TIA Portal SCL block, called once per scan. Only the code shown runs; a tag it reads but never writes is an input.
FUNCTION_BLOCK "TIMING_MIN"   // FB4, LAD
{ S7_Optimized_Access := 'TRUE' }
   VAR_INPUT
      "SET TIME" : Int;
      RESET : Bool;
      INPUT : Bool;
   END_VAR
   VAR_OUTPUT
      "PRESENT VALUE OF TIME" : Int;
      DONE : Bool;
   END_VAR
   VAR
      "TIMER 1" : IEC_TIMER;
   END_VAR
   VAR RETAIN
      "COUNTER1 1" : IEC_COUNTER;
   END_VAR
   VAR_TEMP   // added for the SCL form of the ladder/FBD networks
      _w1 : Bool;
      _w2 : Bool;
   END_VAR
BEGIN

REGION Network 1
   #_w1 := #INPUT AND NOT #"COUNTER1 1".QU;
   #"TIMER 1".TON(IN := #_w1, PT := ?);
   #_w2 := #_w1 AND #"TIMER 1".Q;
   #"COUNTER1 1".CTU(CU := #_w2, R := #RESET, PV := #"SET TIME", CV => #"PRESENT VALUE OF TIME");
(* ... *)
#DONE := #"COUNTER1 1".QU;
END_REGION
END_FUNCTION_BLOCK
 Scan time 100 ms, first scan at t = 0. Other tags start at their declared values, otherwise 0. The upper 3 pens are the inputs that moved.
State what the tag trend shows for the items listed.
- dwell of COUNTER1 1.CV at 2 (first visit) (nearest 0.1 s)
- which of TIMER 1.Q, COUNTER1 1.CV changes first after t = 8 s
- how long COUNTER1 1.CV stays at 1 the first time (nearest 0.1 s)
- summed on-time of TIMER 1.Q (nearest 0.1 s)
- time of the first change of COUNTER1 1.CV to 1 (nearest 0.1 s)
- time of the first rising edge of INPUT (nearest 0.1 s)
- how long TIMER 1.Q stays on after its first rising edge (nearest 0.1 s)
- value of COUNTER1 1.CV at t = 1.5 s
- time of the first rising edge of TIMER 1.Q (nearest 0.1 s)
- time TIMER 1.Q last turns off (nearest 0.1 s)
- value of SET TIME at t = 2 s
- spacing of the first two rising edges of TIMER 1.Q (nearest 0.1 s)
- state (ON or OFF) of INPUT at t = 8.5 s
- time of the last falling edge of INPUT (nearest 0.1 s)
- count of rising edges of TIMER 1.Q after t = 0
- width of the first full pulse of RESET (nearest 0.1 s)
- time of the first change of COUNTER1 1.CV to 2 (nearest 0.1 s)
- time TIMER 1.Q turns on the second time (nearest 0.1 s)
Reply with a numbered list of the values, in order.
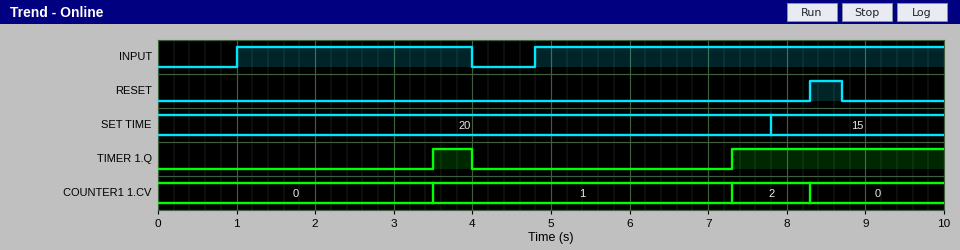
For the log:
1. 1.0 s
2. COUNTER1 1.CV
3. 3.8 s
4. 3.2 s
5. 3.5 s
6. 1.0 s
7. 0.5 s
8. 0
9. 3.5 s
10. 4.0 s
11. 20
12. 3.8 s
13. ON
14. 4.0 s
15. 2
16. 0.4 s
17. 7.3 s
18. 7.3 s
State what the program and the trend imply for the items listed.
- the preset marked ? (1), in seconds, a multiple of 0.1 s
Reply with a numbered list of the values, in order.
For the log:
1. 2.5 s
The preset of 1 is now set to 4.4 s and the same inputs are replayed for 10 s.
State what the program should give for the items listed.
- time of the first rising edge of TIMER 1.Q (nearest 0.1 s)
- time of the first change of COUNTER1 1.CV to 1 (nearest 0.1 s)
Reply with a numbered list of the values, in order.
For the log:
1. 9.2 s
2. 9.2 s
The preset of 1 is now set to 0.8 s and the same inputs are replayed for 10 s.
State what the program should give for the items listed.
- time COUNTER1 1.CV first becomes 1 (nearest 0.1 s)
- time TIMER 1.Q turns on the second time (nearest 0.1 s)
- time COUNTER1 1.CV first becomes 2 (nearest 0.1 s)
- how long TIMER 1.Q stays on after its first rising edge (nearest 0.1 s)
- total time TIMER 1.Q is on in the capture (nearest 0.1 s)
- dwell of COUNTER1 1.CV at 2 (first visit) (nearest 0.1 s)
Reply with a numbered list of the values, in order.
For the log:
1. 1.8 s
2. 5.6 s
3. 5.6 s
4. 2.2 s
5. 6.6 s
6. 2.7 s
